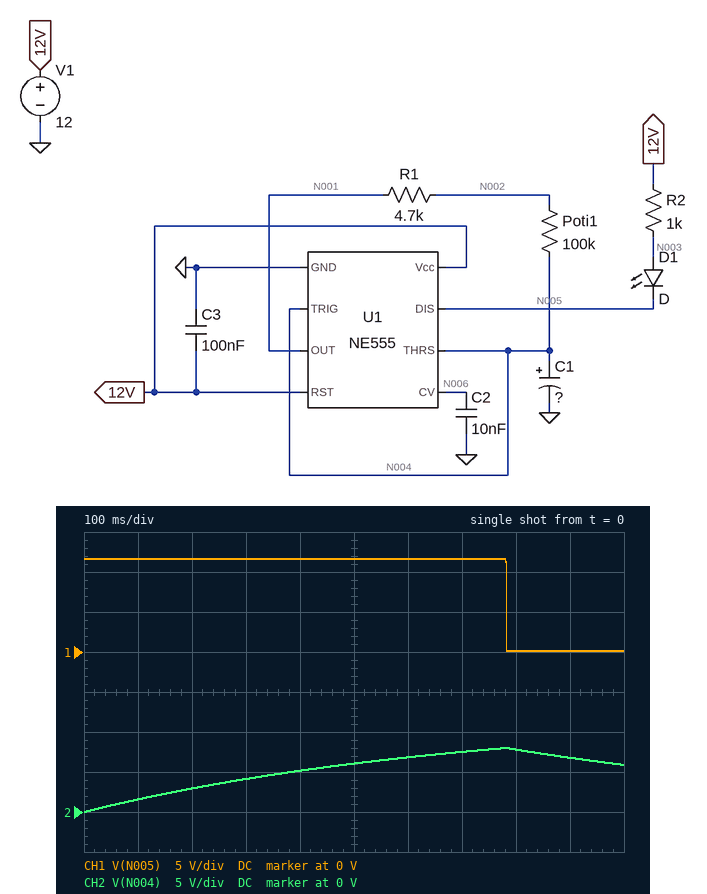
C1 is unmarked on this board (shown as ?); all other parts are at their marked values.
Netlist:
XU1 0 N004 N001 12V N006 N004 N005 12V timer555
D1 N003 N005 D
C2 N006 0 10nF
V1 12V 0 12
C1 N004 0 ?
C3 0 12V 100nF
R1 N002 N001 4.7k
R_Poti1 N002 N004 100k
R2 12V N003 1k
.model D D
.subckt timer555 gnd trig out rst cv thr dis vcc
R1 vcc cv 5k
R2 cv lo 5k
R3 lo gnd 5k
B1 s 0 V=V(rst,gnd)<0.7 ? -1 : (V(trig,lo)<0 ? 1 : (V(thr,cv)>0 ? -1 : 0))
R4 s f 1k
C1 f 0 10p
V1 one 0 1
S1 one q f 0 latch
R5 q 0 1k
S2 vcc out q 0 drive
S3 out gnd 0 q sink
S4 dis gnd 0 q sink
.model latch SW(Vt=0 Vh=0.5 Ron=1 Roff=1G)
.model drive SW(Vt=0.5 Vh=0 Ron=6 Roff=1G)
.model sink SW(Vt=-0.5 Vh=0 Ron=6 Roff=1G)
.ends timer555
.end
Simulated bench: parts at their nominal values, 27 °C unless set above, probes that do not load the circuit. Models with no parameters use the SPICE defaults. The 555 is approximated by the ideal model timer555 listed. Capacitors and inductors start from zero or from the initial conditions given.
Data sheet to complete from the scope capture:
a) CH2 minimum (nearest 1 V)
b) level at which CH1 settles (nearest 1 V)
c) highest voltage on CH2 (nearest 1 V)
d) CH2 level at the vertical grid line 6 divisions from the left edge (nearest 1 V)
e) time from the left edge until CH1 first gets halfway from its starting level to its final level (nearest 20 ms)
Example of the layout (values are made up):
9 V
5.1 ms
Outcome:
0 V
0 V
8 V
7 V
780 ms
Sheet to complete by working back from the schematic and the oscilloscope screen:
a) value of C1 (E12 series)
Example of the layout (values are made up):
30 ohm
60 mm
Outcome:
6.8 µF
